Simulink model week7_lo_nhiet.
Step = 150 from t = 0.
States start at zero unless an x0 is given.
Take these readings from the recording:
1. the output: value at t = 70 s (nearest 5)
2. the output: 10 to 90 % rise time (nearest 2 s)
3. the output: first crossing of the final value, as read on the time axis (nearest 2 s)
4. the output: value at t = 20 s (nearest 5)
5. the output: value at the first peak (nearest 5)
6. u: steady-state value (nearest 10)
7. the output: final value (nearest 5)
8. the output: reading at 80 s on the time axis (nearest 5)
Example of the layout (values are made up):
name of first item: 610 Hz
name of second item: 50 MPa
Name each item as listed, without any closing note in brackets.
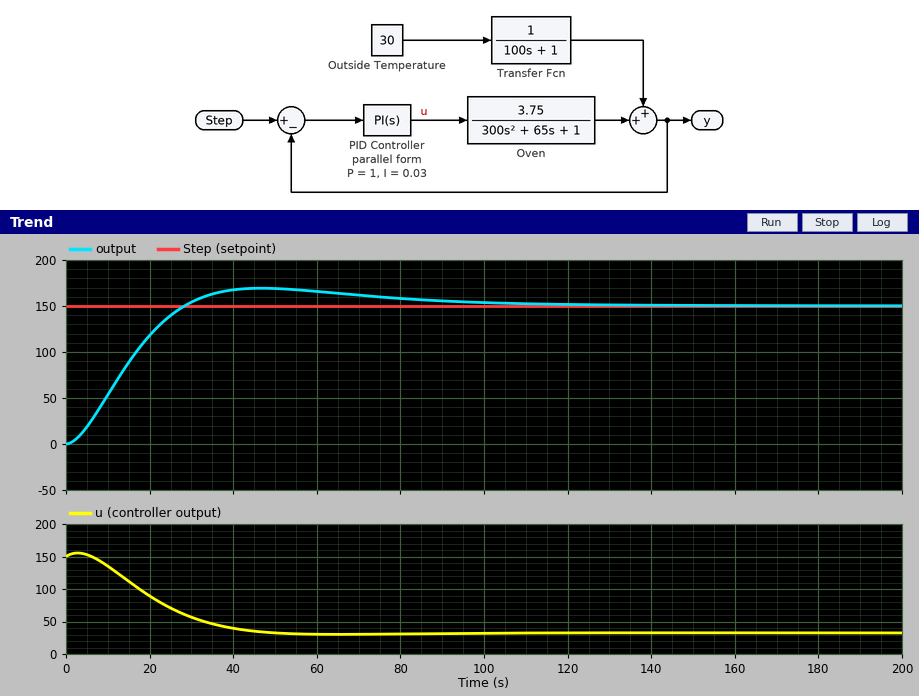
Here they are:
the output: value at t = 70 s: 160
the output: 10 to 90 % rise time: 20 s
the output: first crossing of the final value, as read on the time axis: 28 s
the output: value at t = 20 s: 120
the output: value at the first peak: 170
u: steady-state value: 30
the output: final value: 150
the output: reading at 80 s on the time axis: 160
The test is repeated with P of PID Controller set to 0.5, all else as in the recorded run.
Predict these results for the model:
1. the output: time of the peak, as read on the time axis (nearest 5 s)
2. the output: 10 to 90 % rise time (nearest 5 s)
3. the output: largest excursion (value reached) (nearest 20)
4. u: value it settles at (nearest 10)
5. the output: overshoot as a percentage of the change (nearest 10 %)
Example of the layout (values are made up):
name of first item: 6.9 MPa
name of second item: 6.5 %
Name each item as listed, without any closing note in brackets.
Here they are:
the output: time of the peak, as read on the time axis: 60 s
the output: 10 to 90 % rise time: 25 s
the output: largest excursion (value reached): 200
u: value it settles at: 30
the output: overshoot as a percentage of the change: 30 %
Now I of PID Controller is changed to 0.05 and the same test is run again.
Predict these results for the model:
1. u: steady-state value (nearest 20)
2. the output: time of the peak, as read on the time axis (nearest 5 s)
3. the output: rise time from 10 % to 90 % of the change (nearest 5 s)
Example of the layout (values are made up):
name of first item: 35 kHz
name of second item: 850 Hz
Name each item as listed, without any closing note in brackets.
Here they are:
u: steady-state value: 40
the output: time of the peak, as read on the time axis: 40 s
the output: rise time from 10 % to 90 % of the change: 15 s
